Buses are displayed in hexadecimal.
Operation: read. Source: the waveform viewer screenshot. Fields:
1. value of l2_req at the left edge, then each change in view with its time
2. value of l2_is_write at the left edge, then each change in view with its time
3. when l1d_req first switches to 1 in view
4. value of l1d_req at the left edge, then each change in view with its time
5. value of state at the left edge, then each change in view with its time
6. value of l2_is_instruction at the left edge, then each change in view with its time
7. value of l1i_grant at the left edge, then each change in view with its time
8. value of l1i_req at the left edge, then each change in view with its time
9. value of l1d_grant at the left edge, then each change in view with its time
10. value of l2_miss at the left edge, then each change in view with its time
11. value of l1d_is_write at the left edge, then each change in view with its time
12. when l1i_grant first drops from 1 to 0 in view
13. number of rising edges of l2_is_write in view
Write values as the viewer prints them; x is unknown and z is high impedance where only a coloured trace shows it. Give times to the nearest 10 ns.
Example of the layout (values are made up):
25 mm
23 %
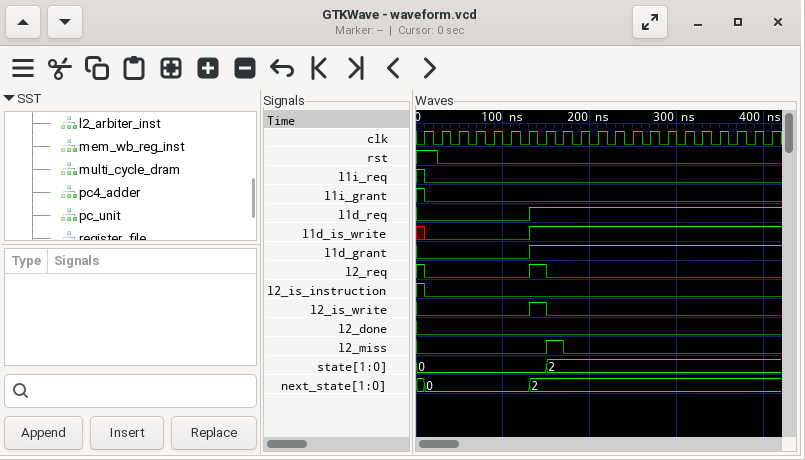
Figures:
1, 0 at 10 ns, 1 at 130 ns, 0 at 150 ns
0, 1 at 130 ns, 0 at 150 ns
130 ns
0, 1 at 130 ns
0, 2 at 150 ns
1, 0 at 10 ns
1, 0 at 10 ns
1, 0 at 10 ns
0, 1 at 130 ns
0, 1 at 150 ns, 0 at 170 ns
x, 0 at 10 ns, 1 at 130 ns
10 ns
1
